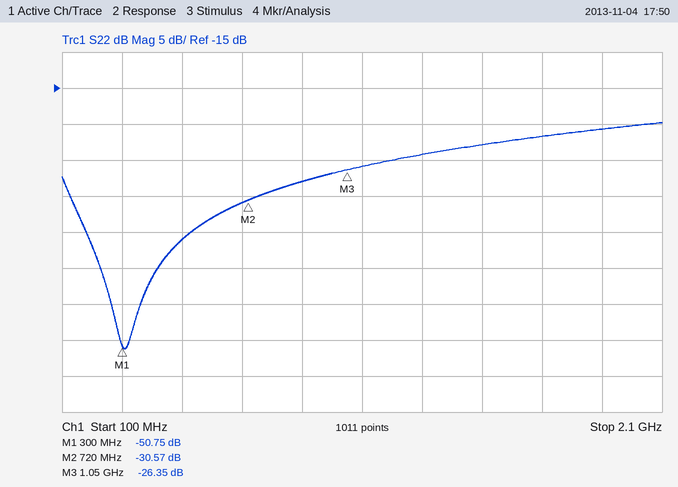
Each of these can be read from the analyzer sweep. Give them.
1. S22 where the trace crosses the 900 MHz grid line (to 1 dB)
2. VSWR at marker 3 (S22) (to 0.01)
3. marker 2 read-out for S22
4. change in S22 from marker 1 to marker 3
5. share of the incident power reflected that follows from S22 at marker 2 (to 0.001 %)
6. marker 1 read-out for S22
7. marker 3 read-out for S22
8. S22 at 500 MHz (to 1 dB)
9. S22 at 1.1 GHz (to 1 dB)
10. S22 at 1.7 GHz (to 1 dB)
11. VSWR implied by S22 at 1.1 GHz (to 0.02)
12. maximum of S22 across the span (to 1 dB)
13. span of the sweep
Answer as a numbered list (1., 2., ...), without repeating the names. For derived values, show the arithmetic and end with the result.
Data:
1. -28 dB
2. (1 + 0.0481)/(1 − 0.0481) ≈ 1.10
3. -30.57 dB
4. -26.35 − (-50.75) = 24.40 dB
5. 10^(-30.57/10) ≈ 0.088 %
6. -50.75 dB
7. -26.35 dB
8. -36 dB
9. -26 dB
10. -22 dB
11. |Γ| = 10^(-26/20) = 0.0501; VSWR = (1 + 0.0501)/(1 − 0.0501) ≈ 1.11, so 1.10 to the nearest 0.02
12. -20 dB
13. 2 GHz
